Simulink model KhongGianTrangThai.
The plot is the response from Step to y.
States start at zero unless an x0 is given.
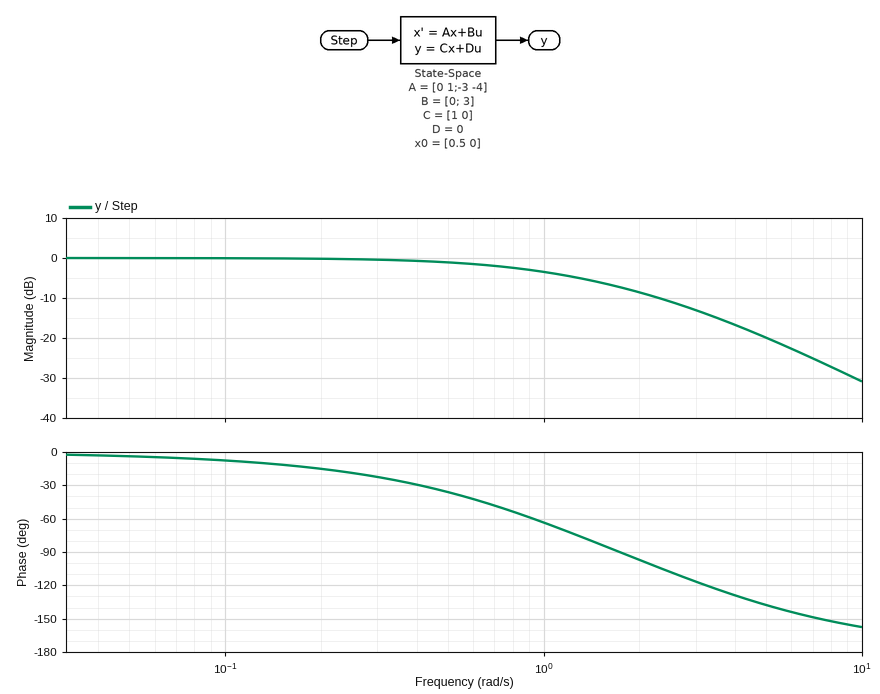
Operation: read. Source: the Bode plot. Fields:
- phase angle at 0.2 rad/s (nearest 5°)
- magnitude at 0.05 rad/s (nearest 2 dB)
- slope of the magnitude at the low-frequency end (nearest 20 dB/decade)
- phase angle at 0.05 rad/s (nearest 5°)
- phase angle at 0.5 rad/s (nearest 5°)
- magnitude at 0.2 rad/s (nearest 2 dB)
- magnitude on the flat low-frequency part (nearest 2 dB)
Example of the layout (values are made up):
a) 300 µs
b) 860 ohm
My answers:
a) -15°
b) 0 dB
c) 0 dB/decade
d) -5°
e) -35°
f) 0 dB
g) 0 dB
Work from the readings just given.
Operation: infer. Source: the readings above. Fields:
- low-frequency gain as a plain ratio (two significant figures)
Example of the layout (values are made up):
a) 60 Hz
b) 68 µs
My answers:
a) 1.0
